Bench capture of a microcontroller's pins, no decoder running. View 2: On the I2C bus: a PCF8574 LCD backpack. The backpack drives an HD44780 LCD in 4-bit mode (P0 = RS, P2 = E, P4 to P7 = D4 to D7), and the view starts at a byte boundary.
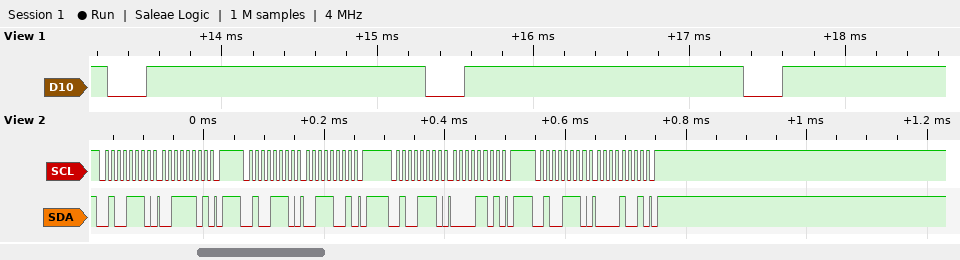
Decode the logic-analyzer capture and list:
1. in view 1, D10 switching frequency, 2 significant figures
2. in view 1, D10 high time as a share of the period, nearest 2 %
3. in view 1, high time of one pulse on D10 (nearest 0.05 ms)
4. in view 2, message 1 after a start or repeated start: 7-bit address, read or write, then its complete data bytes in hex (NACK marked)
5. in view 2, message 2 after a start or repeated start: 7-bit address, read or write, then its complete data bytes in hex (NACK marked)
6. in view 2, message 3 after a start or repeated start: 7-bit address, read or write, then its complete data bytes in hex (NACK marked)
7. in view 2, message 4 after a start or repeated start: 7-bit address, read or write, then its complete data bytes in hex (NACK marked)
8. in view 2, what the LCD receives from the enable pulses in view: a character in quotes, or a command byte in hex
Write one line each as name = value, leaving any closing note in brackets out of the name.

in view 1, D10 switching frequency, 2 significant figures = 490 Hz
in view 1, D10 high time as a share of the period, nearest 2 % = 88 %
in view 1, high time of one pulse on D10 = 1.80 ms
in view 2, message 1 after a start or repeated start: 7-bit address, read or write, then its complete data bytes in hex = 0x27 write: 3D
in view 2, message 2 after a start or repeated start: 7-bit address, read or write, then its complete data bytes in hex = 0x27 write: 39
in view 2, message 3 after a start or repeated start: 7-bit address, read or write, then its complete data bytes in hex = 0x27 write: 0D
in view 2, message 4 after a start or repeated start: 7-bit address, read or write, then its complete data bytes in hex = 0x27 write: 09
in view 2, what the LCD receives from the enable pulses in view: a character in quotes, or a command byte in hex = '0'
